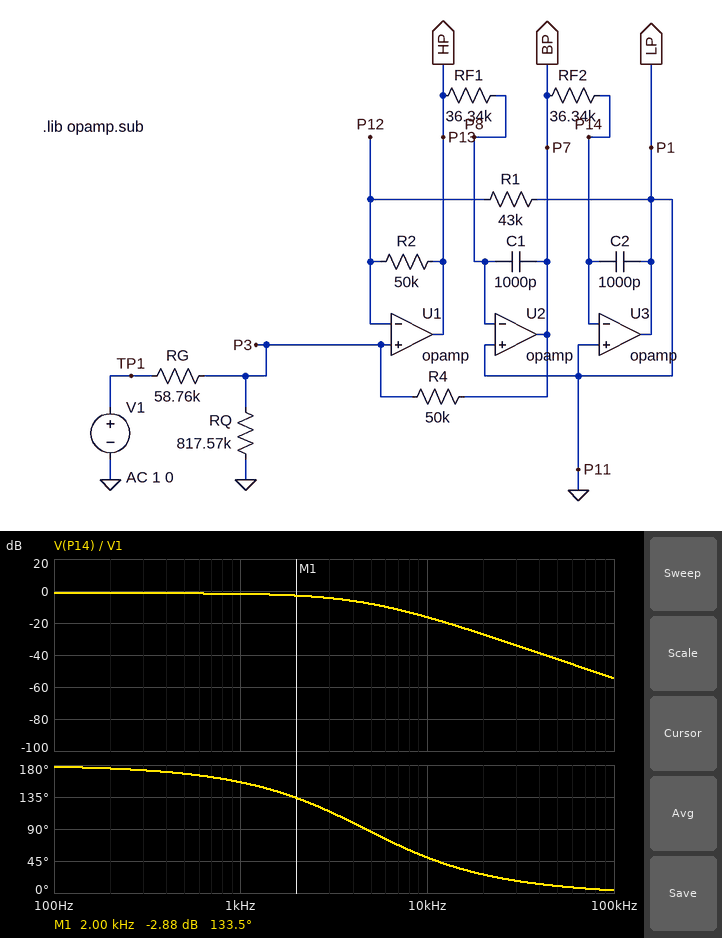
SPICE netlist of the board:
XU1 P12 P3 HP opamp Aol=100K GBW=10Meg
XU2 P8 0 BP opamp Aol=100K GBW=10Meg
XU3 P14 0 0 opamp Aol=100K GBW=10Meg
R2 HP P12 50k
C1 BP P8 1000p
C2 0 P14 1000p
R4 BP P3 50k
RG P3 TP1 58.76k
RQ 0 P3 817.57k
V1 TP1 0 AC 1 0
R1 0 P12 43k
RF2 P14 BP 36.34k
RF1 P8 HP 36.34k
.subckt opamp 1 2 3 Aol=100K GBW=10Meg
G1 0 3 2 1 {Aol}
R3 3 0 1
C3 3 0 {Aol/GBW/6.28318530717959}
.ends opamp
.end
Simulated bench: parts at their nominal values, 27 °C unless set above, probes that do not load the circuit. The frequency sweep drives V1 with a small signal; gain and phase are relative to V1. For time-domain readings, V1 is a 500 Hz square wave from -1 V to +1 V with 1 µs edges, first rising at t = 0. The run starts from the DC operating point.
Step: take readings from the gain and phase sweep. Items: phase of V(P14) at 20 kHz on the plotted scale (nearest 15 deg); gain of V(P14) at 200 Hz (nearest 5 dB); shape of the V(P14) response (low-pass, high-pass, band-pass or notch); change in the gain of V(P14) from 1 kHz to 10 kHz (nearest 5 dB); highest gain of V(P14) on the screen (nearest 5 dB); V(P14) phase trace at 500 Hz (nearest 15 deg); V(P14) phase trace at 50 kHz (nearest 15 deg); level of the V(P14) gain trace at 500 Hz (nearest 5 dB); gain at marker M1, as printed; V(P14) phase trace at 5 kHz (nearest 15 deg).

30 deg
0 dB
low-pass
-15 dB
0 dB
165 deg
15 deg
0 dB
-2.88 dB
90 deg
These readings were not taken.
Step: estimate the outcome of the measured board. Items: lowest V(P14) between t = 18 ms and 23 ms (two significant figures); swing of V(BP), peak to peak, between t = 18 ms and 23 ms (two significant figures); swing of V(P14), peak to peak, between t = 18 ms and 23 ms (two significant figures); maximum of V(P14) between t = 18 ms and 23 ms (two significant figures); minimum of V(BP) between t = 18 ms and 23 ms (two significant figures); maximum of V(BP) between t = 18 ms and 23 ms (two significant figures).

-850 mV
1.7 V
1.7 V
850 mV
-850 mV
850 mV
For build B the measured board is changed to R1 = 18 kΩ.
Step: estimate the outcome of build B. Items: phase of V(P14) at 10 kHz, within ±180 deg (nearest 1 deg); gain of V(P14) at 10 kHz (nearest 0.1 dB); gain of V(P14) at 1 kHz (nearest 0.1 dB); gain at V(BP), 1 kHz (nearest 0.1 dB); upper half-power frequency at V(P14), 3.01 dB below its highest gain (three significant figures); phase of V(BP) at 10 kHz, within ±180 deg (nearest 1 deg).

64 deg
-13.0 dB
-1.7 dB
-1.5 dB
3.66 kHz
131 deg
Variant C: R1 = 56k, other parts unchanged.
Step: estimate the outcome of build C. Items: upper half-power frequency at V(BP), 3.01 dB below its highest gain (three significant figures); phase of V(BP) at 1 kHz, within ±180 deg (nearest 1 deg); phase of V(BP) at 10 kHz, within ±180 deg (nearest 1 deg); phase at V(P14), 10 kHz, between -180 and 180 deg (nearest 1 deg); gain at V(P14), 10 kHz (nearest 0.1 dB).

4.34 kHz
167 deg
113 deg
47 deg
-17.3 dB
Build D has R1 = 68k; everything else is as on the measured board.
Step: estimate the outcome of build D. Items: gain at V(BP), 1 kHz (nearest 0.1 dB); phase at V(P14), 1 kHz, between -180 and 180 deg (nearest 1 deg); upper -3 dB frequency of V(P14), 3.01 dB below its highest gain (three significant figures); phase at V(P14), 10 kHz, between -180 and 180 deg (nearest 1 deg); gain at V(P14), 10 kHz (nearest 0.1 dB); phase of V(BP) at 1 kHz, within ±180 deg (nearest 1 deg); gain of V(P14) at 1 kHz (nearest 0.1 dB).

-1.7 dB
153 deg
2.68 kHz
45 deg
-18.0 dB
166 deg
-1.9 dB
